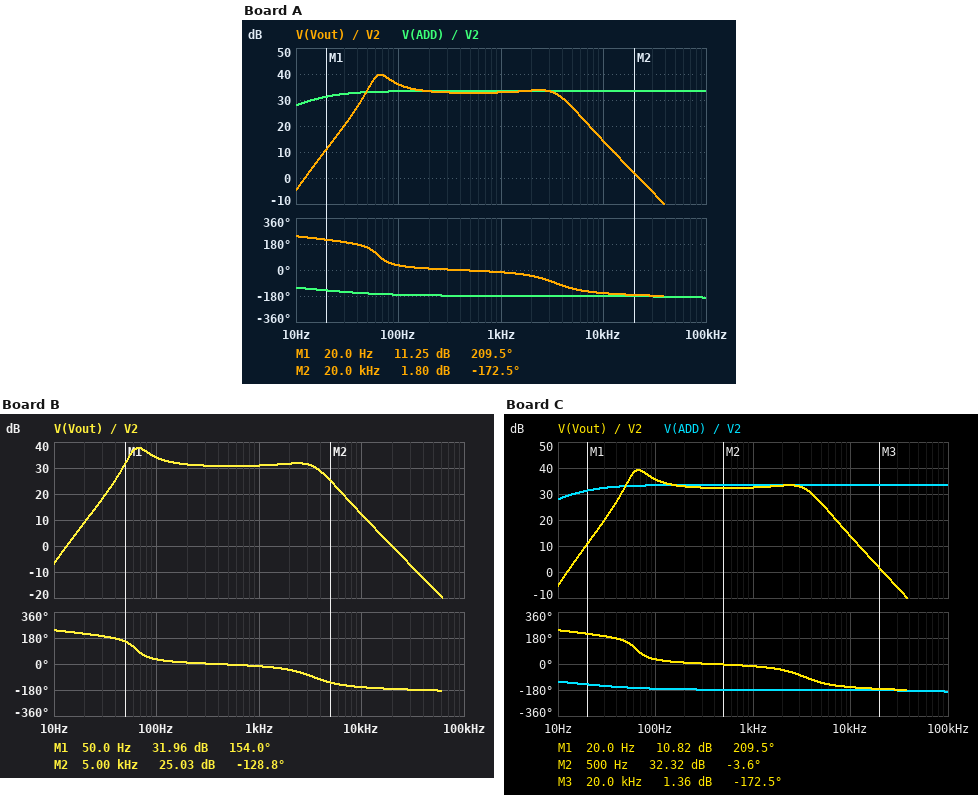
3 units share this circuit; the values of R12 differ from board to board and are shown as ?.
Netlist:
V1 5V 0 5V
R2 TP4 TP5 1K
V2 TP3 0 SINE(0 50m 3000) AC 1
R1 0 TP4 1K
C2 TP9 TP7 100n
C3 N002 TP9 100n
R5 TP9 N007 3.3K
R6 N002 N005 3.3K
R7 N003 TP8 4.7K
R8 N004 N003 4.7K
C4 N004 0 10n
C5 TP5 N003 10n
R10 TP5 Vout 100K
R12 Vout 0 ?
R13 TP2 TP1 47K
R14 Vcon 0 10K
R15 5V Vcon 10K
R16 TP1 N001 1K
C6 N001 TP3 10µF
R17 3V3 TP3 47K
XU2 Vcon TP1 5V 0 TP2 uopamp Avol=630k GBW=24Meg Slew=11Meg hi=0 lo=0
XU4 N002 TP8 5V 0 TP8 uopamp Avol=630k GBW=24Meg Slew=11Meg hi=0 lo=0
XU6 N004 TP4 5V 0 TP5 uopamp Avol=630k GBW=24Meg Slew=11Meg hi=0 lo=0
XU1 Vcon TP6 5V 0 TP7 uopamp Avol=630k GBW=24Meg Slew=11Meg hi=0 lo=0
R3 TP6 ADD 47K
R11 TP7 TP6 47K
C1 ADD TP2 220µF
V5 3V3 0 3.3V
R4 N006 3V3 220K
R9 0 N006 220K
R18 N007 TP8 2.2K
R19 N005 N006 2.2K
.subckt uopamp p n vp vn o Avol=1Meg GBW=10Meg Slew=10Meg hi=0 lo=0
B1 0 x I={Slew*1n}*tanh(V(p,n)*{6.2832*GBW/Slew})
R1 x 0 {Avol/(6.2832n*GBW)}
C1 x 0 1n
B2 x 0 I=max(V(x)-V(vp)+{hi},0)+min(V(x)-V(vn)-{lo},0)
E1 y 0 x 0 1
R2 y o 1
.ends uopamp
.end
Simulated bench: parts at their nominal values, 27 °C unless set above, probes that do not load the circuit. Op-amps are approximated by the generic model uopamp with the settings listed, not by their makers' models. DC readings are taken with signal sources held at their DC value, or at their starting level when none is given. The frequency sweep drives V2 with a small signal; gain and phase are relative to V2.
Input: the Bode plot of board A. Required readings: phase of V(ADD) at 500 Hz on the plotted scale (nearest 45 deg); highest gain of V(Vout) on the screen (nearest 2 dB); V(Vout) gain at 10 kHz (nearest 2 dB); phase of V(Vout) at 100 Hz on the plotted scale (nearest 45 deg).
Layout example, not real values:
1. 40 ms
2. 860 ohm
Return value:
1. -180 deg
2. 40 dB
3. 14 dB
4. 45 deg
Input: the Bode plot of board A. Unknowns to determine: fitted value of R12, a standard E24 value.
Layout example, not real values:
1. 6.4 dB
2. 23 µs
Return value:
1. 82 kΩ
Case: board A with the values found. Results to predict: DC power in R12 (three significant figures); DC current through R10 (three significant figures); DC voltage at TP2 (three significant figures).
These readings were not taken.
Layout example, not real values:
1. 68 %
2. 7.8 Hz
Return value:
1. 27.0 µW
2. 18.1 µA
3. 2.50 V
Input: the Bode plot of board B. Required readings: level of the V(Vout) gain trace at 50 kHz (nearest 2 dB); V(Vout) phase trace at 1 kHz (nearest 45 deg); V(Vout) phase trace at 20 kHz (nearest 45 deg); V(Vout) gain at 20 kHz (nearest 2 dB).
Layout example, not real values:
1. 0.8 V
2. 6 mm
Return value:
1. -16 dB
2. 0 deg
3. -180 deg
4. 0 dB
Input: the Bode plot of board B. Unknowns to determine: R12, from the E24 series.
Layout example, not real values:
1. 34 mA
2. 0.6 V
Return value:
1. 56 kΩ
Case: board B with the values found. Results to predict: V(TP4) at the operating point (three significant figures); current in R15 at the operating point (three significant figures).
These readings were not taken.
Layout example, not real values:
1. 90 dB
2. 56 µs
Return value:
1. 1.65 V
2. 250 µA
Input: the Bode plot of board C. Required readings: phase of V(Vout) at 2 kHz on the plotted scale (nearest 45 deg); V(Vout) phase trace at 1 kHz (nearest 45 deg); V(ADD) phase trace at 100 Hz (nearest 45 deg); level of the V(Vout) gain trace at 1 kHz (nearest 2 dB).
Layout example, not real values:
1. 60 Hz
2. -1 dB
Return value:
1. -45 deg
2. 0 deg
3. -180 deg
4. 32 dB
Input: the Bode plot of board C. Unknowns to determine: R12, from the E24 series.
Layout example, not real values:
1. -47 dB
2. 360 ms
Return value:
1. 75 kΩ
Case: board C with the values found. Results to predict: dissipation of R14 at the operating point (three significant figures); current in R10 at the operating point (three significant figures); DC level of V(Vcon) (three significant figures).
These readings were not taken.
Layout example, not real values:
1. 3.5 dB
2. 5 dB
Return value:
1. 625 µW
2. 18.9 µA
3. 2.50 V
